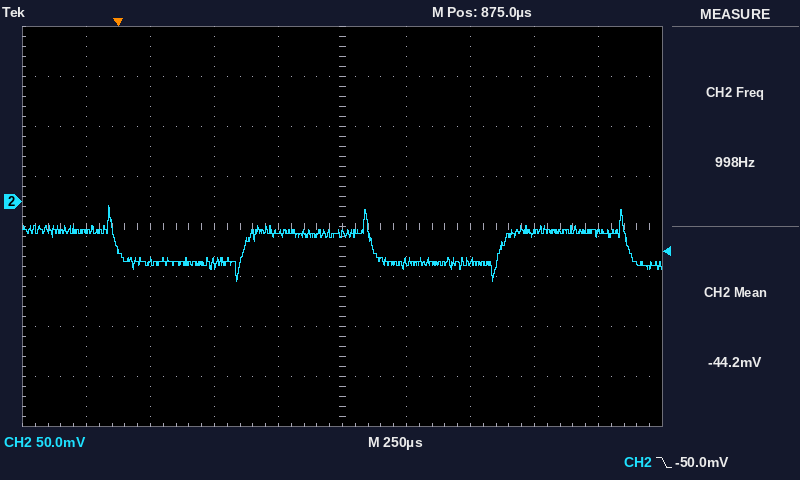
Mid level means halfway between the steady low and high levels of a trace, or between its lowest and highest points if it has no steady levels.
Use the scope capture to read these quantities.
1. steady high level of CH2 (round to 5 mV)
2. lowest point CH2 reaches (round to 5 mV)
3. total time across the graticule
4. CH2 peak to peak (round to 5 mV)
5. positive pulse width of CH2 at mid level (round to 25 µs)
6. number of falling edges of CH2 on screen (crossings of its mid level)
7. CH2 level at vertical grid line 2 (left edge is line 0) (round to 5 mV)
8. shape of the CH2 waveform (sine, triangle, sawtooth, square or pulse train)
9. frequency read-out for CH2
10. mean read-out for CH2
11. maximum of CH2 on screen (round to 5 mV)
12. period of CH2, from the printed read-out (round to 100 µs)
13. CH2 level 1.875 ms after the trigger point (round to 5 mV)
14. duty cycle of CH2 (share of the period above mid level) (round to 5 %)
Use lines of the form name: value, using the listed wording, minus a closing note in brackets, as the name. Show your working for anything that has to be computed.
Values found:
steady high level of CH2: -30 mV
lowest point CH2 reaches: -80 mV
total time across the graticule: 2.5 ms
CH2 peak to peak: -5 mV − (-80 mV) = 75 mV
positive pulse width of CH2 at mid level: 500 µs
number of falling edges of CH2 on screen: 3
CH2 level at vertical grid line 2 (left edge is line 0): -60 mV
shape of the CH2 waveform: square
frequency read-out for CH2: 998 Hz
mean read-out for CH2: -44.2 mV
maximum of CH2 on screen: -5 mV
period of CH2, from the printed read-out: 1 / 998 Hz ≈ 1.0 ms
CH2 level 1.875 ms after the trigger point: -30 mV
duty cycle of CH2 (share of the period above mid level): 50 %
